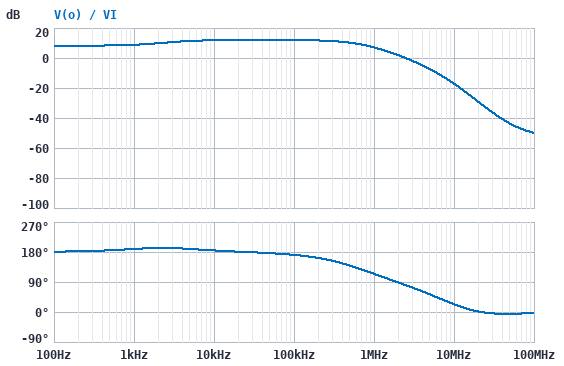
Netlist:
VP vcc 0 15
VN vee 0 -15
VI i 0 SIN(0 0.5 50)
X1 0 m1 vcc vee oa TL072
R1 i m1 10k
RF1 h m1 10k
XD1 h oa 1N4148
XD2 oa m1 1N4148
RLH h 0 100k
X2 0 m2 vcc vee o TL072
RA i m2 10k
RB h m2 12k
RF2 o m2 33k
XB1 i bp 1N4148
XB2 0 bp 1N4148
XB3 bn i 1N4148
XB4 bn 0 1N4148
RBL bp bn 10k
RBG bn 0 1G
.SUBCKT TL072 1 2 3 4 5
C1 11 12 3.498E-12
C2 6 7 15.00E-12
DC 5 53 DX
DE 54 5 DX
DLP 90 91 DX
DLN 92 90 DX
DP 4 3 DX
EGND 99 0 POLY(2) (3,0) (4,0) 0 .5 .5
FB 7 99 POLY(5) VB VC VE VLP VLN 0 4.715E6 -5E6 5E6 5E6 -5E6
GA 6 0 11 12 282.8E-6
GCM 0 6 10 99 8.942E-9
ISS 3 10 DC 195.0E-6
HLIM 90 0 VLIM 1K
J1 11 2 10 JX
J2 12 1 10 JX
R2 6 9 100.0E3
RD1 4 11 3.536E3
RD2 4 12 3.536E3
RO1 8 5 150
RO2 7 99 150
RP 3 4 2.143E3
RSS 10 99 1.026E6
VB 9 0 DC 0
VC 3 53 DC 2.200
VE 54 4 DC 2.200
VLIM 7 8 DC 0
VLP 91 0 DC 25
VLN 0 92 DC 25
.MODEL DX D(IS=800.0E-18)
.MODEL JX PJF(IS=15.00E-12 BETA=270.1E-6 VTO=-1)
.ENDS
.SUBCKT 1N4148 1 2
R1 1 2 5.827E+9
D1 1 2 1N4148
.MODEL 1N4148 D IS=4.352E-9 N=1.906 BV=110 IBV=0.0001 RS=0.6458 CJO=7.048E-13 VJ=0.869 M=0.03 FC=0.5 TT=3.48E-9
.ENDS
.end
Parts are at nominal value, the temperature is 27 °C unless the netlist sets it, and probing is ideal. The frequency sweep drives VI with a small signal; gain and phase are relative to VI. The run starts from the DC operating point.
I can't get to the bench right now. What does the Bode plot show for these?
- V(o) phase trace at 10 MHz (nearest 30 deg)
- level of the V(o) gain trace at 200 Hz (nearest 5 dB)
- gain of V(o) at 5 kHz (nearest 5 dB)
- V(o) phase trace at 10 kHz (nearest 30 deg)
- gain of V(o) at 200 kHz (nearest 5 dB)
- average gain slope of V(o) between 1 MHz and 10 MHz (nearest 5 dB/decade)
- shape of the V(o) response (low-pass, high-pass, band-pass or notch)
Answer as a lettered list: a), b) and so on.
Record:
a) 30 deg
b) 10 dB
c) 10 dB
d) 180 deg
e) 10 dB
f) -25 dB/decade
g) low-pass
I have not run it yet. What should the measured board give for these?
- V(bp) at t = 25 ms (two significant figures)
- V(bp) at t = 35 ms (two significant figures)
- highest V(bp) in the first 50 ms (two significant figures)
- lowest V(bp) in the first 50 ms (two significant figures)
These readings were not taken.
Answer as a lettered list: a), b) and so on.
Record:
a) 250 mV
b) -250 mV
c) 250 mV
d) -250 mV
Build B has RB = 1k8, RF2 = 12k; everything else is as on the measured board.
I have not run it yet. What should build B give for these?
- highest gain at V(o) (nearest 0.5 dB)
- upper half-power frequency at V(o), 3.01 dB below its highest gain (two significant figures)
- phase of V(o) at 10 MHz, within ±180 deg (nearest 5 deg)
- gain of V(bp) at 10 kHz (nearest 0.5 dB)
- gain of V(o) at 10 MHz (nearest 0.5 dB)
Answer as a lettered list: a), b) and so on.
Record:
a) 4.0 dB
b) 1.4 MHz
c) 20 deg
d) -6.0 dB
e) -18.5 dB
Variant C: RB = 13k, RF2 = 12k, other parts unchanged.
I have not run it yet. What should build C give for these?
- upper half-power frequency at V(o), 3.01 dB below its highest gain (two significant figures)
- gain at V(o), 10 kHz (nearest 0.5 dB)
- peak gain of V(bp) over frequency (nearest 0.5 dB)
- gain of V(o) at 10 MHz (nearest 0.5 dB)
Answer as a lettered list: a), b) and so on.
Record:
a) 1.6 MHz
b) 3.0 dB
c) -6.0 dB
d) -19.0 dB
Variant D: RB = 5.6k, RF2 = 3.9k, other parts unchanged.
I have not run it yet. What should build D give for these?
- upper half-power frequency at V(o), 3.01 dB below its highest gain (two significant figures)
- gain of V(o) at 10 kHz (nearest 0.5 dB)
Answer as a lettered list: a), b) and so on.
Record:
a) 3.1 MHz
b) -6.0 dB
